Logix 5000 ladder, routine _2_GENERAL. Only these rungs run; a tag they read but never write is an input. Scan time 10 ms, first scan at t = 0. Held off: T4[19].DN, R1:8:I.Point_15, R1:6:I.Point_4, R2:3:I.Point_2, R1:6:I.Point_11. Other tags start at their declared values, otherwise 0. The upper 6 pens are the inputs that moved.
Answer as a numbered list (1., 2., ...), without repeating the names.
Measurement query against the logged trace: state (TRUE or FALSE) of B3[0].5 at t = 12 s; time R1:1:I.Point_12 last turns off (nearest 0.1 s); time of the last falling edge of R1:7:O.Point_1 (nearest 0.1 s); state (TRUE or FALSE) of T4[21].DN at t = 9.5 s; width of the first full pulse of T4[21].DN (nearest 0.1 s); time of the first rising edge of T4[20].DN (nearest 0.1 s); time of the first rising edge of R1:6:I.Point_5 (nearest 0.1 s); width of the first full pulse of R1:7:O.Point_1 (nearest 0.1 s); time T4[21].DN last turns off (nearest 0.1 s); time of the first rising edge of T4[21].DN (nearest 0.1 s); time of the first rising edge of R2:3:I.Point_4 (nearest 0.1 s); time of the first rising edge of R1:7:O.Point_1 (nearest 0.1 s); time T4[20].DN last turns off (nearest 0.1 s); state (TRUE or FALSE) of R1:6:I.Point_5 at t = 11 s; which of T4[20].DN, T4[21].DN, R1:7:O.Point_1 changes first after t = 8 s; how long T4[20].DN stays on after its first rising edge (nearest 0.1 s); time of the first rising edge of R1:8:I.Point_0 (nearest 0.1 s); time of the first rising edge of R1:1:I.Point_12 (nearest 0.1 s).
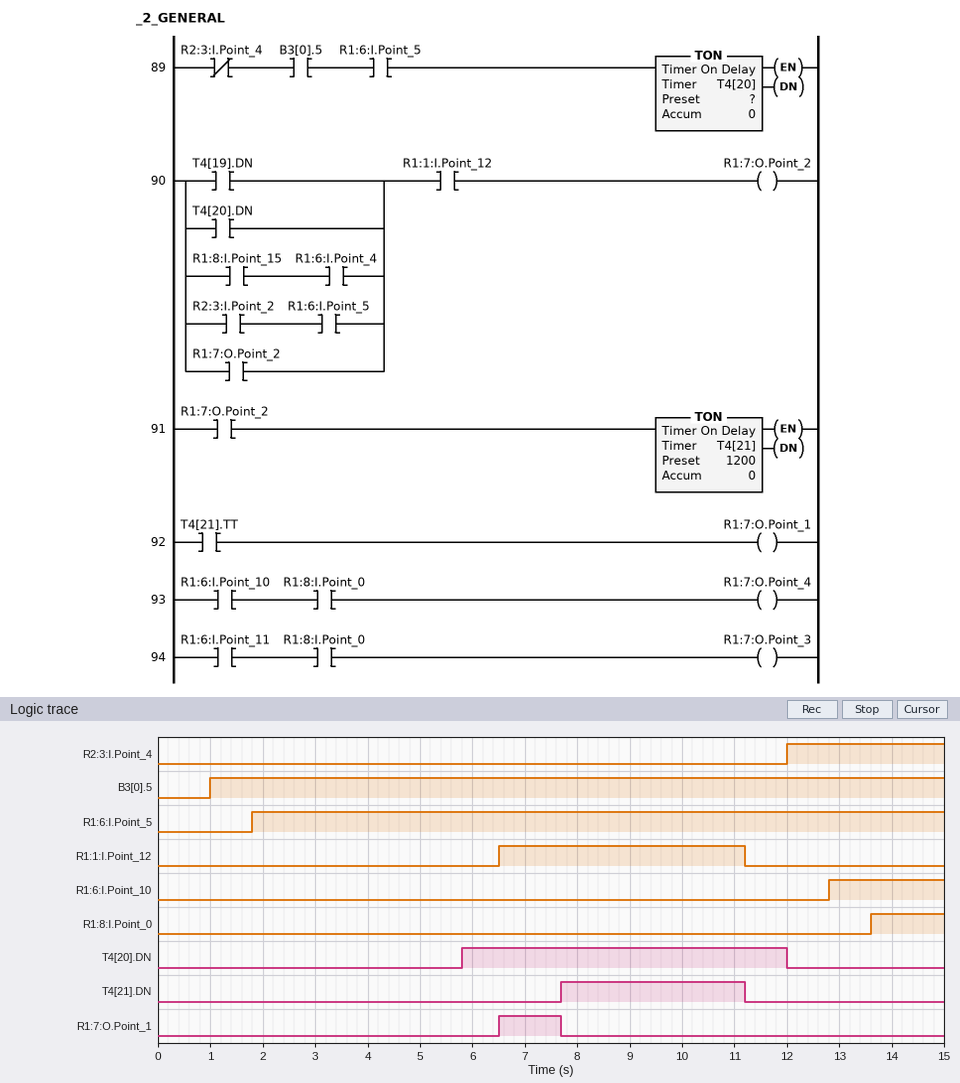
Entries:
1. TRUE
2. 11.2 s
3. 7.7 s
4. TRUE
5. 3.5 s
6. 5.8 s
7. 1.8 s
8. 1.2 s
9. 11.2 s
10. 7.7 s
11. 12.0 s
12. 6.5 s
13. 12.0 s
14. TRUE
15. T4[21].DN
16. 6.2 s
17. 13.6 s
18. 6.5 s
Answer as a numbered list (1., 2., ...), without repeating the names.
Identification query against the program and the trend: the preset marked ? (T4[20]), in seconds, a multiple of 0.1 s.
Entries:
1. 4.0 s
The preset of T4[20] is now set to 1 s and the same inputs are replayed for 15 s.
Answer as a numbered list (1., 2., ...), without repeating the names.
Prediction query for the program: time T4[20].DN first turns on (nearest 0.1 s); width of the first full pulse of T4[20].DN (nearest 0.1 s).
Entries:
1. 2.8 s
2. 9.2 s
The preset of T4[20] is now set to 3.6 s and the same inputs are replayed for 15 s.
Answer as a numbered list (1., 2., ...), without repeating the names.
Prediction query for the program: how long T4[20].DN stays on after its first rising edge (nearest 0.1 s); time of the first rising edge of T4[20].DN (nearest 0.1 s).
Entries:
1. 6.6 s
2. 5.4 s
